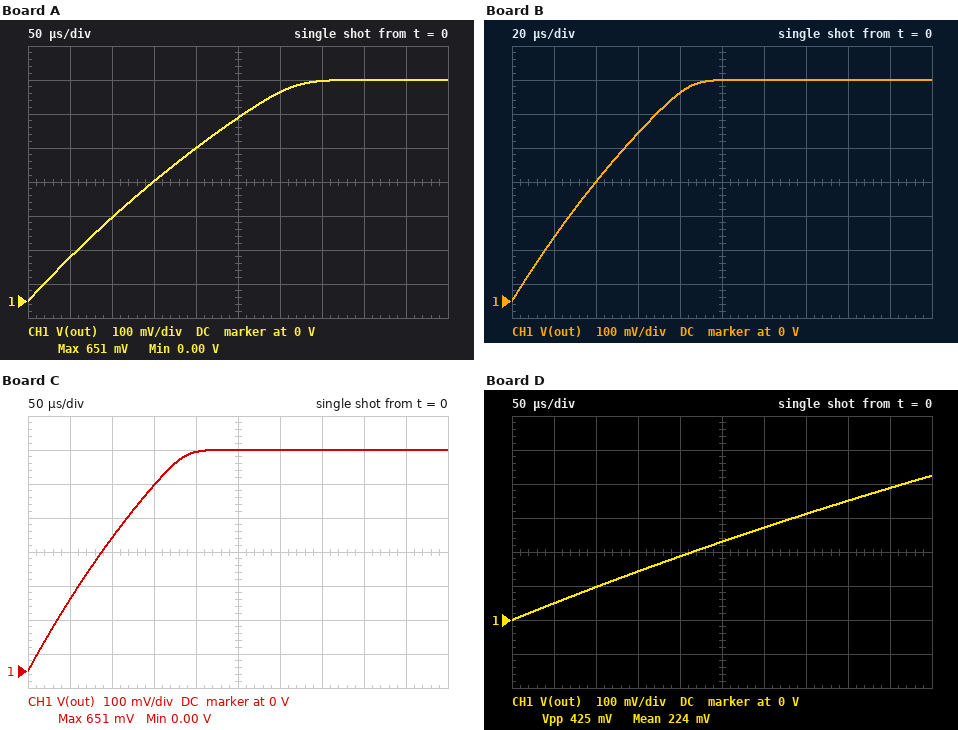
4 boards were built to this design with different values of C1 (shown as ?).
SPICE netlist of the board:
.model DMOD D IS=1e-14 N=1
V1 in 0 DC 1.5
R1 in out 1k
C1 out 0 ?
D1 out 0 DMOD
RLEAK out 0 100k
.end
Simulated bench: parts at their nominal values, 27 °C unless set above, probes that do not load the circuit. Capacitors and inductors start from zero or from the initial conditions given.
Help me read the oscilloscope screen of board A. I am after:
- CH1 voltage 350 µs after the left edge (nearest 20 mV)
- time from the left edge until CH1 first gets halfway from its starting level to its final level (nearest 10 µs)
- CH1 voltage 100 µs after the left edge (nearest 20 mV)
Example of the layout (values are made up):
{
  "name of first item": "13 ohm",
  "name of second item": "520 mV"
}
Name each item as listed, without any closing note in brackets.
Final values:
{
  "CH1 voltage 350 µs after the left edge": "640 mV",
  "time from the left edge until CH1 first gets halfway from its starting level to its final level": "140 µs",
  "CH1 voltage 100 µs after the left edge": "240 mV"
}
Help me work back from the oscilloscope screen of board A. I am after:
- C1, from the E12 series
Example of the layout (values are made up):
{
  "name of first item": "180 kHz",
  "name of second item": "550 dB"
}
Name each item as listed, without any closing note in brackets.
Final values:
{
  "C1, from the E12 series": "560 nF"
}
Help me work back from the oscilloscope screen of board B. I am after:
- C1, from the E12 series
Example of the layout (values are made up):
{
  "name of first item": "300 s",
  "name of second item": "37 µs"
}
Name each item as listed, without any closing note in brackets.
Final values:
{
  "C1, from the E12 series": "150 nF"
}
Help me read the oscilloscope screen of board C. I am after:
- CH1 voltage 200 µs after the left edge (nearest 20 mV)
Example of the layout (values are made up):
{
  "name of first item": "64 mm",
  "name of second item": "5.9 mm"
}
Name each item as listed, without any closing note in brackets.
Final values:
{
  "CH1 voltage 200 µs after the left edge": "640 mV"
}
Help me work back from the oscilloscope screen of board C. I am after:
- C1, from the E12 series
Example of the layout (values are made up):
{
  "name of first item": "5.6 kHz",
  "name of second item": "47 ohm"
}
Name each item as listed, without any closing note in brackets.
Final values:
{
  "C1, from the E12 series": "330 nF"
}
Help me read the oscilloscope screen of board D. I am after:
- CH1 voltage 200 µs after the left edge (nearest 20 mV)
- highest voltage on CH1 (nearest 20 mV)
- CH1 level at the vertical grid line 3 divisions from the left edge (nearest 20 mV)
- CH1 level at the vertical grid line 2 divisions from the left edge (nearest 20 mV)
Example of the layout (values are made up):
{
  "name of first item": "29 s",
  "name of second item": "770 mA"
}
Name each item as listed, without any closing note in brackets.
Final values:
{
  "CH1 voltage 200 µs after the left edge": "180 mV",
  "highest voltage on CH1": "420 mV",
  "CH1 level at the vertical grid line 3 divisions from the left edge": "140 mV",
  "CH1 level at the vertical grid line 2 divisions from the left edge": "100 mV"
}
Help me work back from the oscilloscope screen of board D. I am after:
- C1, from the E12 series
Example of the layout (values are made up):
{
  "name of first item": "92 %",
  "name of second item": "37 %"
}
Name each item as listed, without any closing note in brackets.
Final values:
{
  "C1, from the E12 series": "1.5 µF"
}
